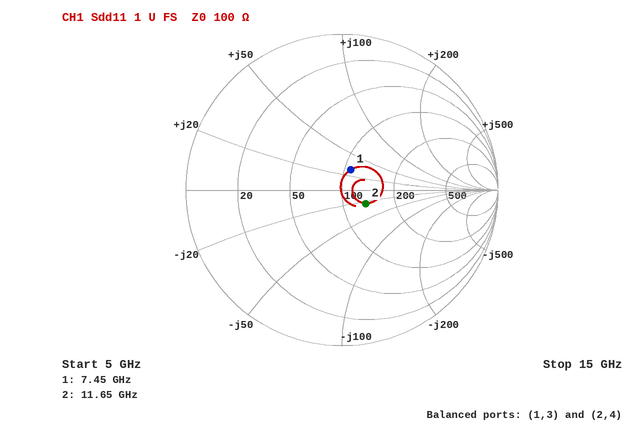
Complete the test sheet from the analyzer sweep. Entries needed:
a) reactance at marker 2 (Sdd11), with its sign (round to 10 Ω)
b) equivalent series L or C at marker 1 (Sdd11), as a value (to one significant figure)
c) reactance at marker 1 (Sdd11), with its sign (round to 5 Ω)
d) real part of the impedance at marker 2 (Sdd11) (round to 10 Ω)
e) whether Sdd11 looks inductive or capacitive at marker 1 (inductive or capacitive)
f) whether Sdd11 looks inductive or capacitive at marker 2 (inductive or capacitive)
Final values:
-20 Ω
600 pH
+30 Ω
130 Ω
inductive
capacitive
